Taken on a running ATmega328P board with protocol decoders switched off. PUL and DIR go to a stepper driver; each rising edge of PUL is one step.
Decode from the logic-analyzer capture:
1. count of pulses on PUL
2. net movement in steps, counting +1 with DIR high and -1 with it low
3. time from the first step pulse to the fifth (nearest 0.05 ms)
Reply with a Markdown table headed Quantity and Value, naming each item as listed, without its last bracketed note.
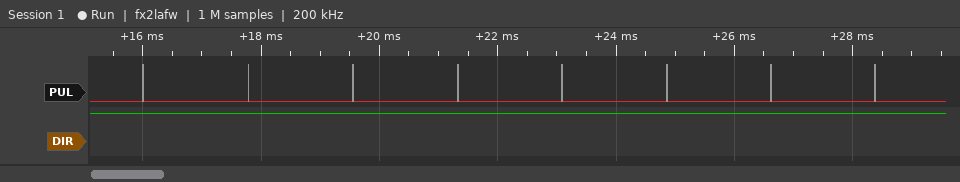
| Quantity | Value |
|---|---|
| count of pulses on PUL | 8 |
| net movement in steps, counting +1 with DIR high and -1 with it low | +8 |
| time from the first step pulse to the fifth | 7.10 ms |
